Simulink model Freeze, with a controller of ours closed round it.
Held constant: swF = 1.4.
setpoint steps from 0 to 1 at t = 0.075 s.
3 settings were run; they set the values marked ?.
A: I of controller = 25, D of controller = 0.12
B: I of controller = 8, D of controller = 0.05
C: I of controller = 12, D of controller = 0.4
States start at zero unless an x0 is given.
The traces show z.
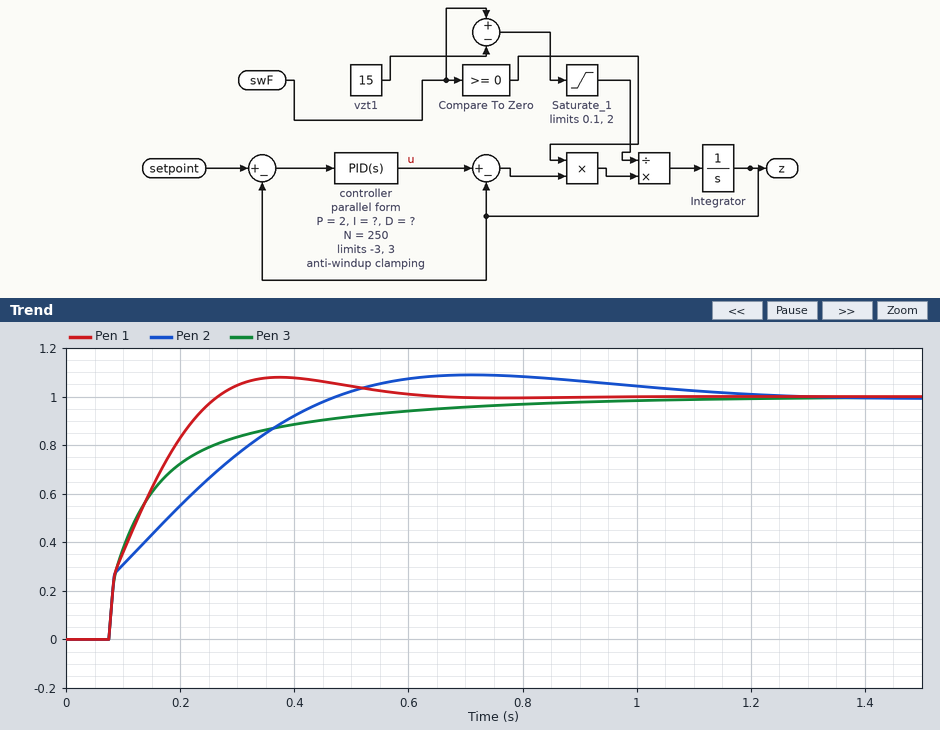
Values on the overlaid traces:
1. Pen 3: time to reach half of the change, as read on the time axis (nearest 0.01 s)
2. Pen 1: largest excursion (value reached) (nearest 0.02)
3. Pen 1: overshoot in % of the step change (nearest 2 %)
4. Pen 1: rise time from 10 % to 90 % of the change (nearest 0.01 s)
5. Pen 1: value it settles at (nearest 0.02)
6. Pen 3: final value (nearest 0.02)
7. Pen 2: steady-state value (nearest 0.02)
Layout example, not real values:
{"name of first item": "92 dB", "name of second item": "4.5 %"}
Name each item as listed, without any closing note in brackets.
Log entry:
{"Pen 3: time to reach half of the change, as read on the time axis": "0.12 s", "Pen 1: largest excursion (value reached)": "1.08", "Pen 1: overshoot in % of the step change": "8 %", "Pen 1: rise time from 10 % to 90 % of the change": "0.14 s", "Pen 1: value it settles at": "1.00", "Pen 3: final value": "1.00", "Pen 2: steady-state value": "1.00"}
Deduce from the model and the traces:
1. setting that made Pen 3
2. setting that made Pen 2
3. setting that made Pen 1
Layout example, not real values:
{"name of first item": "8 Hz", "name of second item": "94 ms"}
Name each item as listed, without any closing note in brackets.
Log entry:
{"setting that made Pen 3": "B", "setting that made Pen 2": "C", "setting that made Pen 1": "A"}
